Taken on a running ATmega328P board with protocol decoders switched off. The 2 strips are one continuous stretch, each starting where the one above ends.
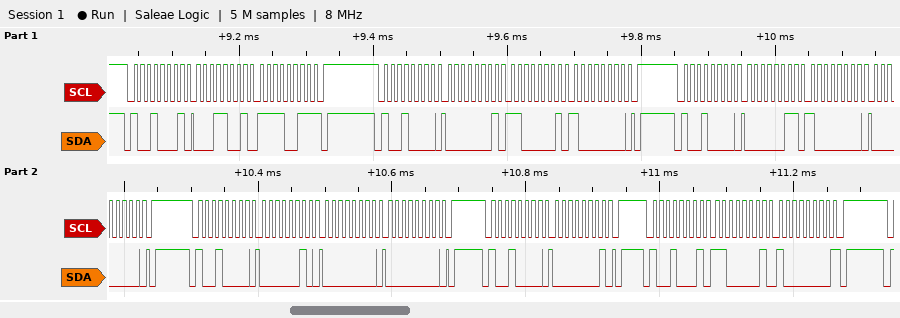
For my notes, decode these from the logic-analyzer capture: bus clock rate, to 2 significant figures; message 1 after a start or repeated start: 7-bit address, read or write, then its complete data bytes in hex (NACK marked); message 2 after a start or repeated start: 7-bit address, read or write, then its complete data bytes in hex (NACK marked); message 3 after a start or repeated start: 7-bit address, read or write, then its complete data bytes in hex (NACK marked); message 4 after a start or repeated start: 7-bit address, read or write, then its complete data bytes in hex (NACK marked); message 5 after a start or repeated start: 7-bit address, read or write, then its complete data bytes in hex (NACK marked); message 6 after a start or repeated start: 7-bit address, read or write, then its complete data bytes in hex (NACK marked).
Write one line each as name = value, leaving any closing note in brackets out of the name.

bus clock rate, to 2 significant figures = 100 kHz
message 1 after a start or repeated start: 7-bit address, read or write, then its complete data bytes in hex = 0x48 read: 19 F3 NACK
message 2 after a start or repeated start: 7-bit address, read or write, then its complete data bytes in hex = 0x48 write: 01 C1 80
message 3 after a start or repeated start: 7-bit address, read or write, then its complete data bytes in hex = 0x48 write: 03 80 00
message 4 after a start or repeated start: 7-bit address, read or write, then its complete data bytes in hex = 0x48 write: 02 00 00
message 5 after a start or repeated start: 7-bit address, read or write, then its complete data bytes in hex = 0x48 write: 01
message 6 after a start or repeated start: 7-bit address, read or write, then its complete data bytes in hex = 0x48 read: C1 80 NACK
